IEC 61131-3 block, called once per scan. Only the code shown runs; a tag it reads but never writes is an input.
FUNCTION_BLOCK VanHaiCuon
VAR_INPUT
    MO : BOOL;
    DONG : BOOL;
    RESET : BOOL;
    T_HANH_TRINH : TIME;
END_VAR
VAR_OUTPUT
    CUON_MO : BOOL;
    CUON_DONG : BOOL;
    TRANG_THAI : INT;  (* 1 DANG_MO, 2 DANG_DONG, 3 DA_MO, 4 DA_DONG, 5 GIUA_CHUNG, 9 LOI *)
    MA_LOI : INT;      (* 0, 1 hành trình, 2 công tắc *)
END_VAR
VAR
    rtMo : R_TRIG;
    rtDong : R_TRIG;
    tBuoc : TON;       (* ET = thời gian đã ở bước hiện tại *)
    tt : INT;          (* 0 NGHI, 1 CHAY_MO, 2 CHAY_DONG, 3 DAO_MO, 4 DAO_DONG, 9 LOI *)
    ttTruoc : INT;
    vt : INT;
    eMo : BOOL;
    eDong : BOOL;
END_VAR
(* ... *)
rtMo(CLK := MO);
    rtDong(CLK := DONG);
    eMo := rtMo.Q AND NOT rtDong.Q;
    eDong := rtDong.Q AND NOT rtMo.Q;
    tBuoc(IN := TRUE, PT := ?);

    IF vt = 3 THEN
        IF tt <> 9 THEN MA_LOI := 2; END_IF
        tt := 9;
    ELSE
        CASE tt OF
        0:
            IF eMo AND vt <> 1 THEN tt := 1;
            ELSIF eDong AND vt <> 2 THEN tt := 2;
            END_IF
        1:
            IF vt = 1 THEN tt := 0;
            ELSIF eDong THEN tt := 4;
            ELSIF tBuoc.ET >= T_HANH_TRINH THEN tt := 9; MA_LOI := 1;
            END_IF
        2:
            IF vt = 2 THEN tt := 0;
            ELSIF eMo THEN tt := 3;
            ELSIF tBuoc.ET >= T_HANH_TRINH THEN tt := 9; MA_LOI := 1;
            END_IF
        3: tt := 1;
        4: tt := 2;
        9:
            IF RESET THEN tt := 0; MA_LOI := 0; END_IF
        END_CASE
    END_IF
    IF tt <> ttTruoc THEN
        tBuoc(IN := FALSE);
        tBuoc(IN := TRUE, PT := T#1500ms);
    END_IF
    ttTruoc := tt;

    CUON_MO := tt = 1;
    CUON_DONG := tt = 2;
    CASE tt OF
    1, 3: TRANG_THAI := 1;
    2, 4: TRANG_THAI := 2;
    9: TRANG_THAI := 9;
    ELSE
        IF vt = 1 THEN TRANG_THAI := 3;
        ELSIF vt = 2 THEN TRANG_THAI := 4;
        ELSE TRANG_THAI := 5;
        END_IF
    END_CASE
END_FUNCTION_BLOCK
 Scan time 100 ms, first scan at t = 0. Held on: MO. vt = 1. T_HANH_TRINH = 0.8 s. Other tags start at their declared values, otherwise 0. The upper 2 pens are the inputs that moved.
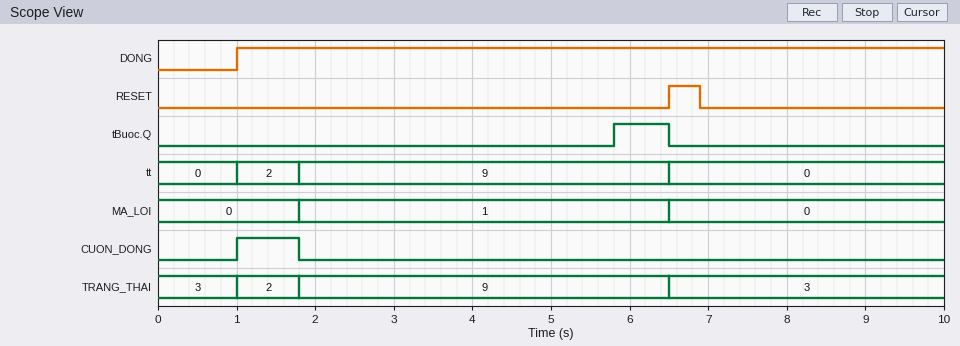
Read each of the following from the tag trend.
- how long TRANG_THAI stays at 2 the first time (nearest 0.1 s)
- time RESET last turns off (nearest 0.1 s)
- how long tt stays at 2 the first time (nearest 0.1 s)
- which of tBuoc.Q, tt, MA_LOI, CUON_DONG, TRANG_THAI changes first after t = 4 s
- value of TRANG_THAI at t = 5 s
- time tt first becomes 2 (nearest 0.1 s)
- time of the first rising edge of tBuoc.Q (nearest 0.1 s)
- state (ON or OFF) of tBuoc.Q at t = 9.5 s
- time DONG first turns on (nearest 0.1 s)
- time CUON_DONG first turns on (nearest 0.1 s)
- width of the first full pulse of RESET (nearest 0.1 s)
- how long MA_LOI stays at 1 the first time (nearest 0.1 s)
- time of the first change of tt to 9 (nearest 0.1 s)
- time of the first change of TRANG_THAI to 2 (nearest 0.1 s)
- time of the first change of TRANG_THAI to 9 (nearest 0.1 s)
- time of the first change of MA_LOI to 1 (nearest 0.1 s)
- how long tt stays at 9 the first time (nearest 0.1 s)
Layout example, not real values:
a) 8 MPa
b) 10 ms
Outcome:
a) 0.8 s
b) 6.9 s
c) 0.8 s
d) tBuoc.Q
e) 9
f) 1.0 s
g) 5.8 s
h) OFF
i) 1.0 s
j) 1.0 s
k) 0.4 s
l) 4.7 s
m) 1.8 s
n) 1.0 s
o) 1.8 s
p) 1.8 s
q) 4.7 s
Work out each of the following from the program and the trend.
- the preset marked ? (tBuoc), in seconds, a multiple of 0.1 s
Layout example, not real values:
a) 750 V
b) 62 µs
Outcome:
a) 4.0 s
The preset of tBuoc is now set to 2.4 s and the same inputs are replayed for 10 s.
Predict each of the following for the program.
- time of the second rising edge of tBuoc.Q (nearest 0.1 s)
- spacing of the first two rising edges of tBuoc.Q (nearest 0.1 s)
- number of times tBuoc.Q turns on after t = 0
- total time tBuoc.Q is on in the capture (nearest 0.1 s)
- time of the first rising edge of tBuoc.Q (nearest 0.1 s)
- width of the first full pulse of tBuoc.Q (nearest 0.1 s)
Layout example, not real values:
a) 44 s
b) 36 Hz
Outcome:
a) 8.9 s
b) 4.7 s
c) 2
d) 3.4 s
e) 4.2 s
f) 2.3 s
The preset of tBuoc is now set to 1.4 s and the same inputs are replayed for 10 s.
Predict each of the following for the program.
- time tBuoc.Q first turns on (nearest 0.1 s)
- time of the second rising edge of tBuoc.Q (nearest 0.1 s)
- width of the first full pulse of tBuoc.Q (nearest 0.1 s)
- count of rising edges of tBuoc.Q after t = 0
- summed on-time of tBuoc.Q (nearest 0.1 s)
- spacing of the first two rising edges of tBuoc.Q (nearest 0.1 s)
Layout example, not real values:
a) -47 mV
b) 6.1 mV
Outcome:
a) 3.2 s
b) 7.9 s
c) 3.3 s
d) 2
e) 5.4 s
f) 4.7 s
